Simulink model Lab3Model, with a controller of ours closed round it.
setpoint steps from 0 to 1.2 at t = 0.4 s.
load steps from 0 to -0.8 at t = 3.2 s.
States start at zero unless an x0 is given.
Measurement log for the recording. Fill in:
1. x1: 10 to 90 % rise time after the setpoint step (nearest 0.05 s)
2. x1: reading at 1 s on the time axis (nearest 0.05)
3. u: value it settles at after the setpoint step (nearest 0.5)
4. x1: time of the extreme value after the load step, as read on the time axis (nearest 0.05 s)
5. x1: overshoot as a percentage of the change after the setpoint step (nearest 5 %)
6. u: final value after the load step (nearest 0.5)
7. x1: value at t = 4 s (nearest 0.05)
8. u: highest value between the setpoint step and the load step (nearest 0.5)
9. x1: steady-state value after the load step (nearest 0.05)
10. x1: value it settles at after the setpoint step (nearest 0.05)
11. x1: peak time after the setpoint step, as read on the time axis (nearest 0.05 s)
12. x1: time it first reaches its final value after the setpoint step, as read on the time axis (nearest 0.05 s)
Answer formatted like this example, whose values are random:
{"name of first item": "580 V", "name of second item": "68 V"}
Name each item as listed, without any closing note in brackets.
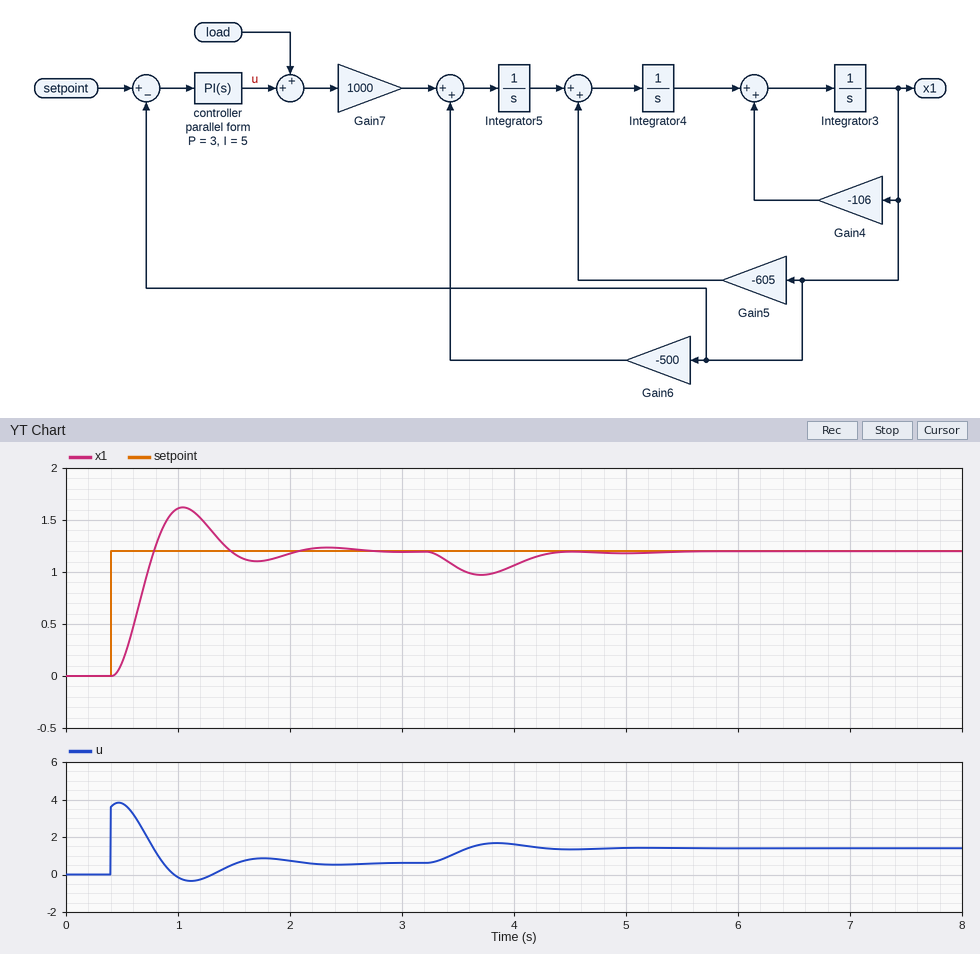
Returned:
{"x1: 10 to 90 % rise time after the setpoint step": "0.25 s", "x1: reading at 1 s on the time axis": "1.60", "u: value it settles at after the setpoint step": "0.5", "x1: time of the extreme value after the load step, as read on the time axis": "3.70 s", "x1: overshoot as a percentage of the change after the setpoint step": "35 %", "u: final value after the load step": "1.5", "x1: value at t = 4 s": "1.05", "u: highest value between the setpoint step and the load step": "4.0", "x1: steady-state value after the load step": "1.20", "x1: value it settles at after the setpoint step": "1.20", "x1: peak time after the setpoint step, as read on the time axis": "1.05 s", "x1: time it first reaches its final value after the setpoint step, as read on the time axis": "0.80 s"}
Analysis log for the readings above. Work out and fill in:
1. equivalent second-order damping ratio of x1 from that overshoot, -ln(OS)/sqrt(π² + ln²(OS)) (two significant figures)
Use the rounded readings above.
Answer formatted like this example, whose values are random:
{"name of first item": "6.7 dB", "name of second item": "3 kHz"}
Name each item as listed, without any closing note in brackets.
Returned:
{"equivalent second-order damping ratio of x1 from that overshoot, -ln(OS)/sqrt(π² + ln²(OS))": "0.32"}
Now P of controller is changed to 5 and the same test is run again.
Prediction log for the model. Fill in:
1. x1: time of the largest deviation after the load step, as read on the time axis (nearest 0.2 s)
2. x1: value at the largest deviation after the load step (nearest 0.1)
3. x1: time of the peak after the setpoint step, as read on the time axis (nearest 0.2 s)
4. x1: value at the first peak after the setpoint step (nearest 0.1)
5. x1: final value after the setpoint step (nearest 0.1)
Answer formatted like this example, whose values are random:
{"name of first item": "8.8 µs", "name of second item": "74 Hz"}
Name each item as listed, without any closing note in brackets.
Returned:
{"x1: time of the largest deviation after the load step, as read on the time axis": "3.6 s", "x1: value at the largest deviation after the load step": "1.0", "x1: time of the peak after the setpoint step, as read on the time axis": "0.8 s", "x1: value at the first peak after the setpoint step": "1.6", "x1: final value after the setpoint step": "1.2"}
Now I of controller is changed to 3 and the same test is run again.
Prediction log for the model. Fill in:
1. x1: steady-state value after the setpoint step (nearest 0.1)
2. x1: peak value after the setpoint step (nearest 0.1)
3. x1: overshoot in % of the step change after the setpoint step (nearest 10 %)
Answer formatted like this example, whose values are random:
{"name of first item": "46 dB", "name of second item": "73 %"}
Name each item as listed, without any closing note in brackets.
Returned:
{"x1: steady-state value after the setpoint step": "1.2", "x1: peak value after the setpoint step": "1.5", "x1: overshoot in % of the step change after the setpoint step": "20 %"}
